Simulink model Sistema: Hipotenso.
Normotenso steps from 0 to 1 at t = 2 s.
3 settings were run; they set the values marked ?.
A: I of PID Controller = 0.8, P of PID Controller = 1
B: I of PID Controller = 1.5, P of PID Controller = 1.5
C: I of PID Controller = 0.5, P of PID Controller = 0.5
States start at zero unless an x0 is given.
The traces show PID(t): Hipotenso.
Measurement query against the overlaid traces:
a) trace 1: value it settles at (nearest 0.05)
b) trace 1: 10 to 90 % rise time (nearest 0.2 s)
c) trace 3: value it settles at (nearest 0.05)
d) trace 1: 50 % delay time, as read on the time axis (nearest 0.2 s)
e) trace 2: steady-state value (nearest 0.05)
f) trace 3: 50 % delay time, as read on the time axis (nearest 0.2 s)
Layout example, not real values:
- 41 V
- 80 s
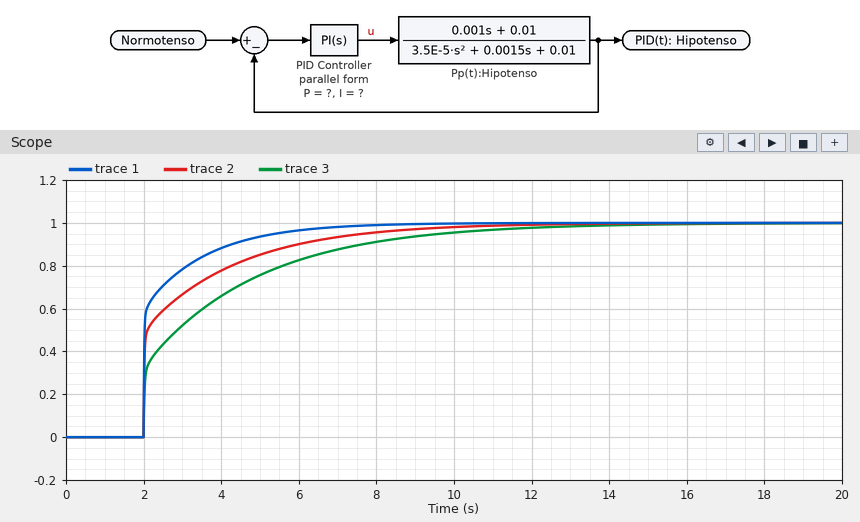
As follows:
- 1.00
- 2.2 s
- 1.00
- 2.0 s
- 1.00
- 2.8 s
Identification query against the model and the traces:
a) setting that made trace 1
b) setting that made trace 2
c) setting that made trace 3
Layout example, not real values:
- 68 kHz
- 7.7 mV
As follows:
- B
- A
- C
